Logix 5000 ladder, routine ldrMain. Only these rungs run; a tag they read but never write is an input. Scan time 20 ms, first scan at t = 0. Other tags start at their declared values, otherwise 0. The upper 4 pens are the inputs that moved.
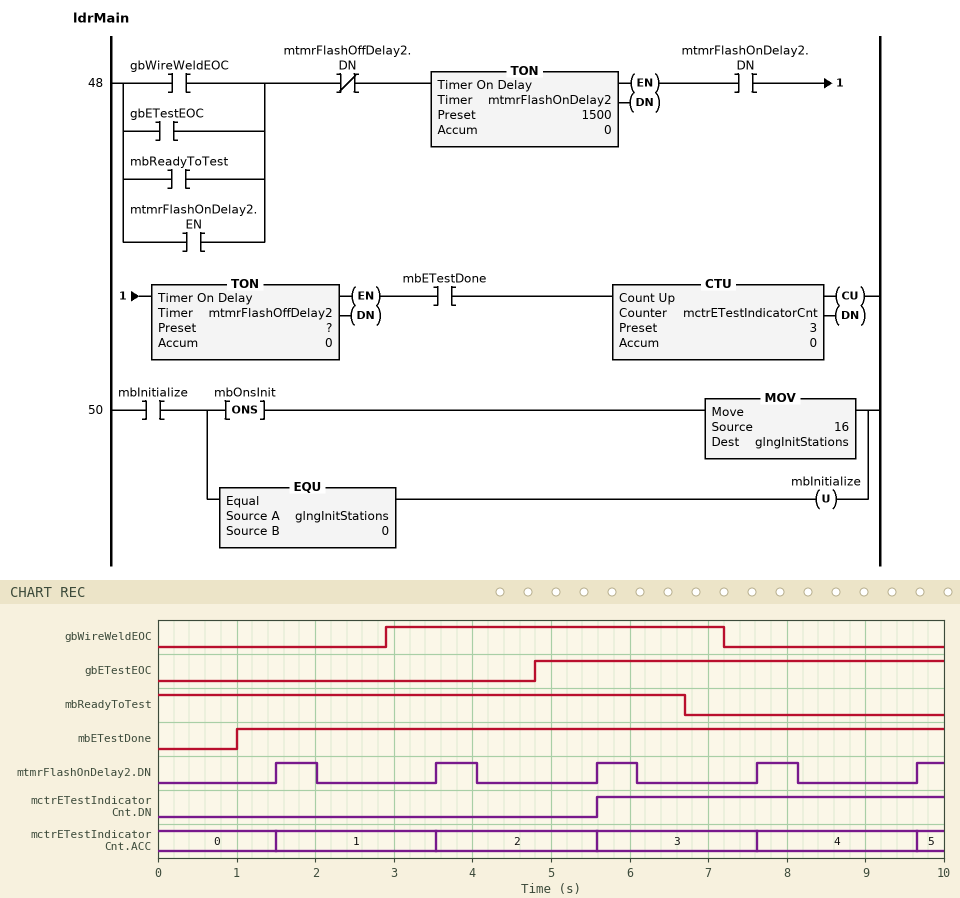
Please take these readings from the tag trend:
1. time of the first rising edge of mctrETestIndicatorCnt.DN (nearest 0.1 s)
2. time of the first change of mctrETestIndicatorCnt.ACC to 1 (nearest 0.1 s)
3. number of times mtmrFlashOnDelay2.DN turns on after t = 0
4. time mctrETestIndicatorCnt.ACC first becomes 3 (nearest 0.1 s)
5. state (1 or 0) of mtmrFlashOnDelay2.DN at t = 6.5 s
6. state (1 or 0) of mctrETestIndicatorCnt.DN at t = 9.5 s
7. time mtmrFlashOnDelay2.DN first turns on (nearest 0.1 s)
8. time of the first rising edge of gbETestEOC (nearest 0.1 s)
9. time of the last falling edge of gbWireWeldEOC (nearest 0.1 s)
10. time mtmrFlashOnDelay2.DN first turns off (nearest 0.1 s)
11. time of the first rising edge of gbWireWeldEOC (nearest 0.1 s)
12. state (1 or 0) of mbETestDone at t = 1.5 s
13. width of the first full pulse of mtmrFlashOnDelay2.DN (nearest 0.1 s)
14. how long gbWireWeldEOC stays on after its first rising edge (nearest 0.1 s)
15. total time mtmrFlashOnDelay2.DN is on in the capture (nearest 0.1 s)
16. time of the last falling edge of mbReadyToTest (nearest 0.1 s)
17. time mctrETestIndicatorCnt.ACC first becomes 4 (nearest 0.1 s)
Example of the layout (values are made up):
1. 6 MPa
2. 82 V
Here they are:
1. 5.6 s
2. 1.5 s
3. 5
4. 5.6 s
5. 0
6. 1
7. 1.5 s
8. 4.8 s
9. 7.2 s
10. 2.0 s
11. 2.9 s
12. 1
13. 0.5 s
14. 4.3 s
15. 2.4 s
16. 6.7 s
17. 7.6 s
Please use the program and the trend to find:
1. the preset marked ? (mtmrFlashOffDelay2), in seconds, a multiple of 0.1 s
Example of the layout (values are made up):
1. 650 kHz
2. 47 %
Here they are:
1. 0.5 s
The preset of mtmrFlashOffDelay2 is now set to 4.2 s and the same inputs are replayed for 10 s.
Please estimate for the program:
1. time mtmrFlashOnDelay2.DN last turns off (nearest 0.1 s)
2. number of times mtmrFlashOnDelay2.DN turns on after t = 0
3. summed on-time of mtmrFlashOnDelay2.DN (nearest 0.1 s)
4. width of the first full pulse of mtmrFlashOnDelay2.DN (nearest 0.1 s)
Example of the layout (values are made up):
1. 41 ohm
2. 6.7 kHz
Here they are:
1. 5.7 s
2. 2
3. 7.0 s
4. 4.2 s
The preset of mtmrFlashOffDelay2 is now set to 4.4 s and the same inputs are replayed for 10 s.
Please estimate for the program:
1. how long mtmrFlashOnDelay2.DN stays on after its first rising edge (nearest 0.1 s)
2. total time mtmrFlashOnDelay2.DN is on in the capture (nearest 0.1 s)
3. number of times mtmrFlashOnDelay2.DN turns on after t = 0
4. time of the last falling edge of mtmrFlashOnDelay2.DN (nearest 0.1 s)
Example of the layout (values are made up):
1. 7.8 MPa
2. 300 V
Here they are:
1. 4.4 s
2. 7.0 s
3. 2
4. 5.9 s
